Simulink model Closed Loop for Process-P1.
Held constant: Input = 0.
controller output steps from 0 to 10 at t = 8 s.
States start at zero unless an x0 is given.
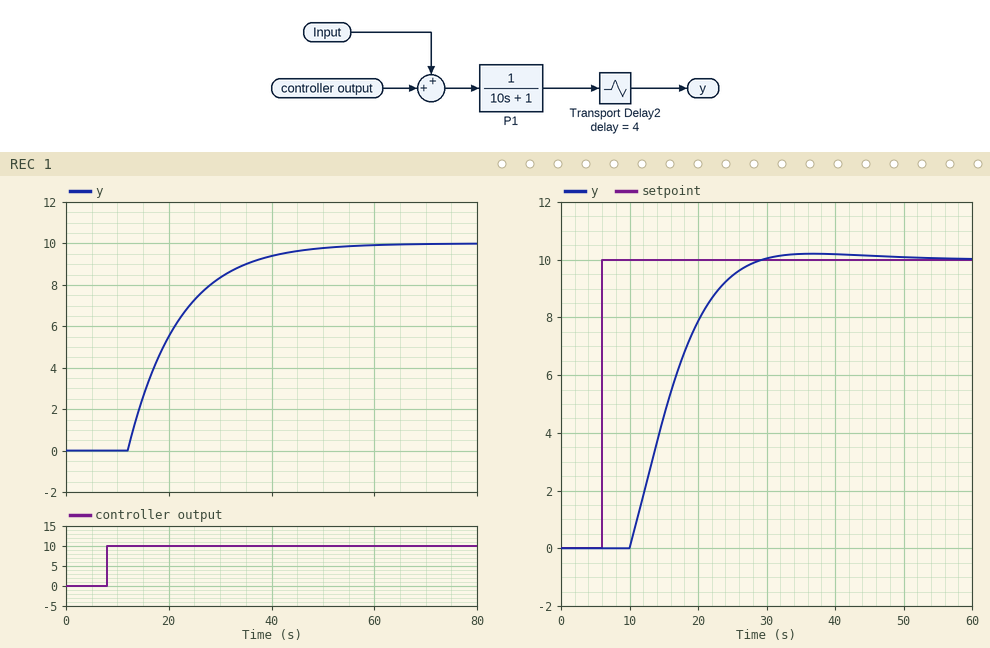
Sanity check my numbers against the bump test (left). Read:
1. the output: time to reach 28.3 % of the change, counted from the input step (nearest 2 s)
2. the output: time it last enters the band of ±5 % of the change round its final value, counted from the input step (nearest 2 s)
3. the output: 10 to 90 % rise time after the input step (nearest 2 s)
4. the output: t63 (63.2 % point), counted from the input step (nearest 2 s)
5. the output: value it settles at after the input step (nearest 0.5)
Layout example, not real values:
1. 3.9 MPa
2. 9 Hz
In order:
1. 8 s
2. 34 s
3. 22 s
4. 14 s
5. 10.0
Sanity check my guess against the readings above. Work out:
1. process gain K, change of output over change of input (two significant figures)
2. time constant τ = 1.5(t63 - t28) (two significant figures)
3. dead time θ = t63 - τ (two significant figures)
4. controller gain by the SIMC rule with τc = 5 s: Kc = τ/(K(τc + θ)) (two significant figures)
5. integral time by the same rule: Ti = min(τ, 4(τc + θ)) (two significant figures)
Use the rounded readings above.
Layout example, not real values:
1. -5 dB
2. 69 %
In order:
1. 1.0
2. 9.0 s
3. 5.0 s
4. 0.90
5. 9.0 s
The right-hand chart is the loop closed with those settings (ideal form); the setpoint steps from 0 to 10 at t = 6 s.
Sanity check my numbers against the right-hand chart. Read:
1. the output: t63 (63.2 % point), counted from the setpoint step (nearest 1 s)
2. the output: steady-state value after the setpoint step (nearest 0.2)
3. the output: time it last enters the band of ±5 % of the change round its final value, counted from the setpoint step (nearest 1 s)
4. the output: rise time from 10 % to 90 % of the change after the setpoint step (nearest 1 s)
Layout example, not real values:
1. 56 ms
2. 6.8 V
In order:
1. 11 s
2. 10.0
3. 19 s
4. 12 s
